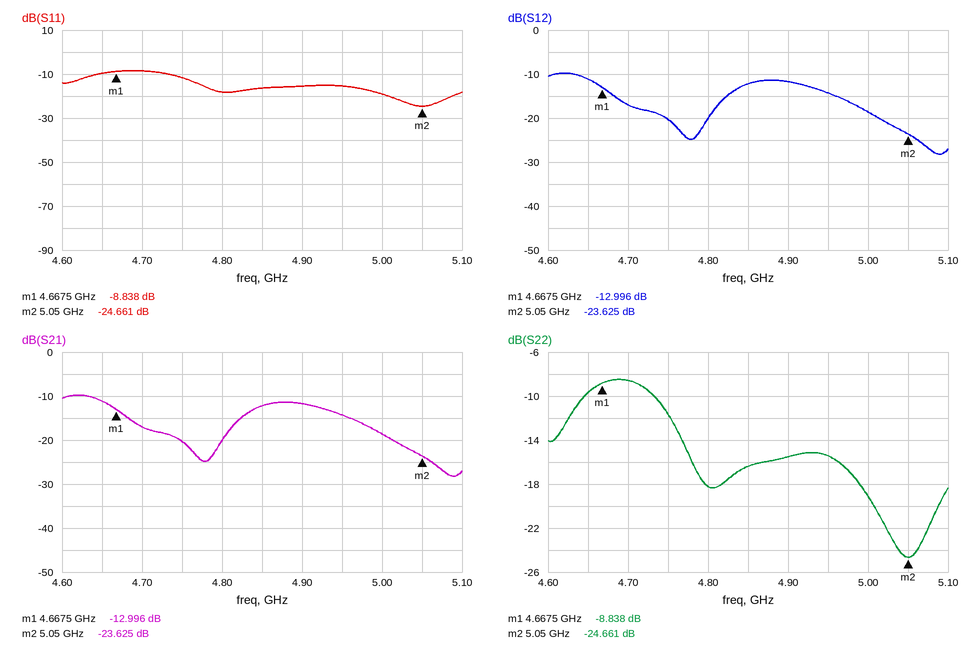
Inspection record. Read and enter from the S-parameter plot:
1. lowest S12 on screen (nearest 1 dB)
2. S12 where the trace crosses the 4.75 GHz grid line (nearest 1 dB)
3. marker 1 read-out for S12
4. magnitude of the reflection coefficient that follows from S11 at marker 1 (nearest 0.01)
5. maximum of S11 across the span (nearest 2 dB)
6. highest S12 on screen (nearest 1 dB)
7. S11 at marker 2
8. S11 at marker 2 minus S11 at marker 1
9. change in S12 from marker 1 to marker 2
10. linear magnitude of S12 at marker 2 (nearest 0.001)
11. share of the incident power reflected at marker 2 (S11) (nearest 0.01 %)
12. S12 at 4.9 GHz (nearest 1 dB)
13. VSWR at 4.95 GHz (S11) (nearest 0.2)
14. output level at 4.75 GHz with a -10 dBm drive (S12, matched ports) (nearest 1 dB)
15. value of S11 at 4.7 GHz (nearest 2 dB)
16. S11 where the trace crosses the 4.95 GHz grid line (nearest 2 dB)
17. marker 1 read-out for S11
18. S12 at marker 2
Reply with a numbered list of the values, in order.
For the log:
1. -28 dB
2. -20 dB
3. -12.996 dB
4. 0.36
5. -8 dB
6. -10 dB
7. -24.661 dB
8. -15.823 dB
9. -10.629 dB
10. 0.066
11. 0.34 %
12. -12 dB
13. 1.4
14. -30 dBm
15. -8 dB
16. -16 dB
17. -8.838 dB
18. -23.625 dB
